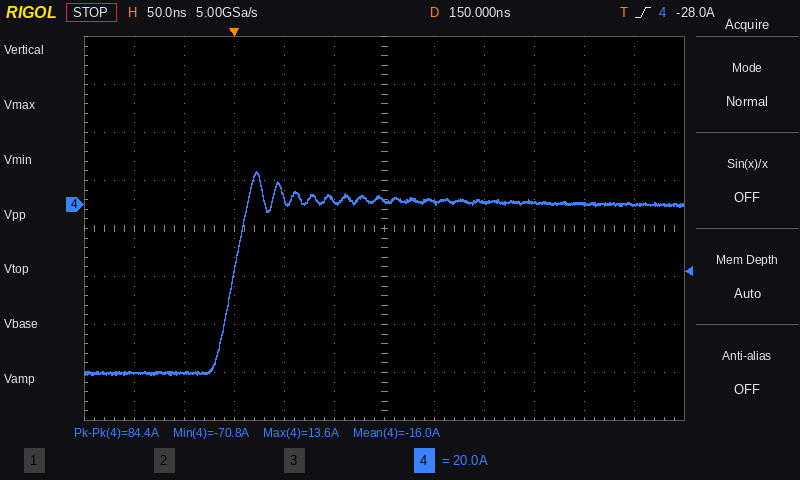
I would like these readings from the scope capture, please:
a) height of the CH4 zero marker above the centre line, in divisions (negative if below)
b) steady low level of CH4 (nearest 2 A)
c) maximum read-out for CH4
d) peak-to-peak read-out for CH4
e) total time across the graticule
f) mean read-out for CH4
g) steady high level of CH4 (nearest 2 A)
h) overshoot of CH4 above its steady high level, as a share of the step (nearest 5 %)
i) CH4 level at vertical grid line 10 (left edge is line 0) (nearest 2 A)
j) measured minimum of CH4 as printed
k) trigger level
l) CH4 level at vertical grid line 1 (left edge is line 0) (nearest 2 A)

+0.5 div
-70 A
13.6 A
84.4 A
600 ns
-16.0 A
0 A
20 %
0 A
-70.8 A
-28.0 A
-70 A
